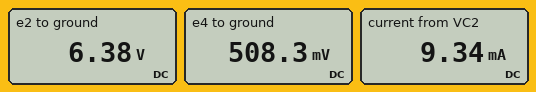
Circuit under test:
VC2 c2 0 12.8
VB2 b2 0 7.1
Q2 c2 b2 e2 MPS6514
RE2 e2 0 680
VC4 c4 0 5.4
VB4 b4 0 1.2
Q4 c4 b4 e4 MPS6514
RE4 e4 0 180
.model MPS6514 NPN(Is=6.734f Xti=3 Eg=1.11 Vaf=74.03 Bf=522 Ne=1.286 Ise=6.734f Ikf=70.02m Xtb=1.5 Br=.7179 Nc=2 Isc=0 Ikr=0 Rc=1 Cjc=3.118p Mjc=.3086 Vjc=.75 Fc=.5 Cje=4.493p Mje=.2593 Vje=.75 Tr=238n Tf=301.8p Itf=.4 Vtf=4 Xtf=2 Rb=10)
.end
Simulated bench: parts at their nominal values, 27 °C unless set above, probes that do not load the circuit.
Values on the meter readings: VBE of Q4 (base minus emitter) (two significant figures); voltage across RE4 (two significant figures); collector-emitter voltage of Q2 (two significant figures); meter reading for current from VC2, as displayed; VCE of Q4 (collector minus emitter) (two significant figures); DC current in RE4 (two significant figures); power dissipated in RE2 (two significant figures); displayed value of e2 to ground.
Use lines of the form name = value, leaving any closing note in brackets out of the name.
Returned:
VBE of Q4 (base minus emitter) = 690 mV
voltage across RE4 = 510 mV
collector-emitter voltage of Q2 = 6.4 V
meter reading for current from VC2, as displayed = 9.34 mA
VCE of Q4 (collector minus emitter) = 4.9 V
DC current in RE4 = 2.8 mA
power dissipated in RE2 = 60 mW
displayed value of e2 to ground = 6.38 V
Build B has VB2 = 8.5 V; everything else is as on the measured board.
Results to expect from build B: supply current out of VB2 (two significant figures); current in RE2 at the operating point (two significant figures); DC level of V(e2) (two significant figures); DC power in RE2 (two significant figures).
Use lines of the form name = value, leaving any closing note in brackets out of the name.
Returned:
supply current out of VB2 = 47 µA
current in RE2 at the operating point = 11 mA
DC level of V(e2) = 7.8 V
DC power in RE2 = 89 mW
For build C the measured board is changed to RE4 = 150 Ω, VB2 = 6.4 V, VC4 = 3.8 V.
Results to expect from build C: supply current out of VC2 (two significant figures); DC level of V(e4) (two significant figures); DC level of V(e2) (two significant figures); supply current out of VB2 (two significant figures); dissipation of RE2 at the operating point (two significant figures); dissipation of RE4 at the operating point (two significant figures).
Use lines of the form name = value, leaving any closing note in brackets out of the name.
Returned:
supply current out of VC2 = 8.3 mA
DC level of V(e4) = 500 mV
DC level of V(e2) = 5.7 V
supply current out of VB2 = 34 µA
dissipation of RE2 at the operating point = 47 mW
dissipation of RE4 at the operating point = 1.7 mW
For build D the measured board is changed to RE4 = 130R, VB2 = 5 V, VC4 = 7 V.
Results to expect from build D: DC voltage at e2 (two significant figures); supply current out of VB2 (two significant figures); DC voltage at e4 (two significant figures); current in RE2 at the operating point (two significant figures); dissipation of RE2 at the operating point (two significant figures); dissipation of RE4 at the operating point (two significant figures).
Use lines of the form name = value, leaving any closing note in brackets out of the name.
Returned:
DC voltage at e2 = 4.3 V
supply current out of VB2 = 25 µA
DC voltage at e4 = 500 mV
current in RE2 at the operating point = 6.3 mA
dissipation of RE2 at the operating point = 27 mW
dissipation of RE4 at the operating point = 1.9 mW
